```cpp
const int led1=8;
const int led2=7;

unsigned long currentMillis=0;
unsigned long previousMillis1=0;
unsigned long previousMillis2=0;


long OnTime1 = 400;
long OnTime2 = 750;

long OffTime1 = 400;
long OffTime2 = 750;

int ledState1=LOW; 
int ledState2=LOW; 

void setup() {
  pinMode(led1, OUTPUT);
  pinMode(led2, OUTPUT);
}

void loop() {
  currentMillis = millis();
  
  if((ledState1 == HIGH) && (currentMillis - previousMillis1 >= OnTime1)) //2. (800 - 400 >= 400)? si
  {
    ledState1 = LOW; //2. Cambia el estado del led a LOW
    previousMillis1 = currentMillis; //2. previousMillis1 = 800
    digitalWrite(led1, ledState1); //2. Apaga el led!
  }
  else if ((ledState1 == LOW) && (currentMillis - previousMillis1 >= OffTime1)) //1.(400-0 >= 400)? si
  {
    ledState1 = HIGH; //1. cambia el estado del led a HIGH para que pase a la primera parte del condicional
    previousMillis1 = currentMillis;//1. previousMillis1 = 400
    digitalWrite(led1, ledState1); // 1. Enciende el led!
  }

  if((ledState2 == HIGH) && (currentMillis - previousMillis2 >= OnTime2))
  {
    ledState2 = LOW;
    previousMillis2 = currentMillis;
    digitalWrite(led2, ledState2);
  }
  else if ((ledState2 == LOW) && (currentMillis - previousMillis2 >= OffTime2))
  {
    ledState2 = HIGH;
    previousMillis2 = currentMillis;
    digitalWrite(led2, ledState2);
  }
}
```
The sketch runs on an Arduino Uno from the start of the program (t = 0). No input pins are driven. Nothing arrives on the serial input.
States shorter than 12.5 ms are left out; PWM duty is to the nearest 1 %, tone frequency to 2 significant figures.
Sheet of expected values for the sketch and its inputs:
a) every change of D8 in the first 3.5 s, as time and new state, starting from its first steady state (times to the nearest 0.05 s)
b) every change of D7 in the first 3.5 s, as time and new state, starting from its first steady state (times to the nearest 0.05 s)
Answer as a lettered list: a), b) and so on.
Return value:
a) 0 s low; 0.4 s high; 0.8 s low; 1.2 s high; 1.6 s low; 2 s high; 2.4 s low; 2.8 s high; 3.2 s low
b) 0 s low; 0.75 s high; 1.5 s low; 2.25 s high; 3 s low
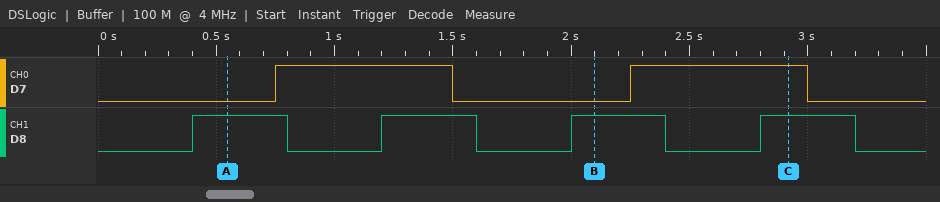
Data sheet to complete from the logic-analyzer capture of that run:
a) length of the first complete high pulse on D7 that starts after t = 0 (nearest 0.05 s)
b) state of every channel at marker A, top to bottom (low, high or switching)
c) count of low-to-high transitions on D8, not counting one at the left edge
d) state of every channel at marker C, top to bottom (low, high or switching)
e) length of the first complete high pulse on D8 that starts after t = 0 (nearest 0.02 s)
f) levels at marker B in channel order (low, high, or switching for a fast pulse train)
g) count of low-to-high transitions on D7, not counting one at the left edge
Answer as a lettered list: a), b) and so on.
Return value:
a) 0.75 s
b) D7 low, D8 high
c) 4
d) D7 high, D8 high
e) 0.40 s
f) D7 low, D8 high
g) 2
